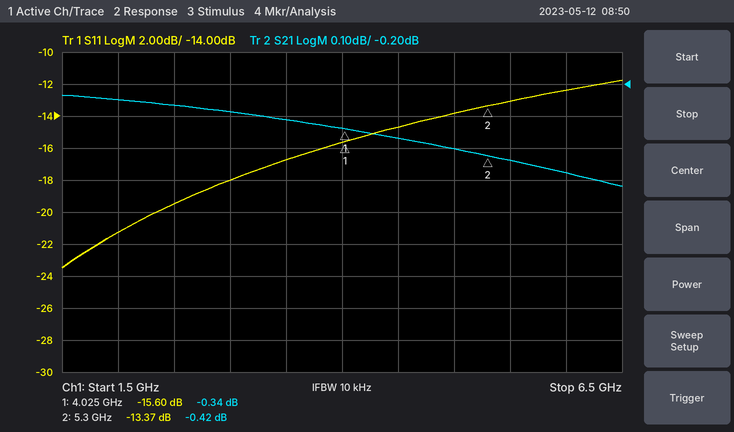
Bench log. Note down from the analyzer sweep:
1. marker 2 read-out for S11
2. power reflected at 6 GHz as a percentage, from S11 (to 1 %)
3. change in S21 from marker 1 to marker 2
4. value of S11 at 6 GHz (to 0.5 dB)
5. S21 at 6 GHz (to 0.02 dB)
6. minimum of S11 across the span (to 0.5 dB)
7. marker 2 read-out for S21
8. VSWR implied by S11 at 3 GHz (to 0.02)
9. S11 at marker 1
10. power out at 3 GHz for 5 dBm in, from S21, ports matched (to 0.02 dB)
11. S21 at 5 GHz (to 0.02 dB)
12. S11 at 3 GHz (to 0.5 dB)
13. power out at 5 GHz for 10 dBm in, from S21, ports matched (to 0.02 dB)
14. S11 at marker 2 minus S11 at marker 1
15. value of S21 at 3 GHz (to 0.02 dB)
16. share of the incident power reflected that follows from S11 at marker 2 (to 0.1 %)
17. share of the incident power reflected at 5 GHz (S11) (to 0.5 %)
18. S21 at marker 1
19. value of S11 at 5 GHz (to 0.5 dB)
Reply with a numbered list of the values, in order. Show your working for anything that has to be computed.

1. -13.37 dB
2. 10^(-12.5/10) ≈ 6 %
3. -0.42 − (-0.34) = -0.08 dB
4. -12.5 dB
5. -0.48 dB
6. -23.5 dB
7. -0.42 dB
8. |Γ| = 10^(-18/20) = 0.1259; VSWR = (1 + 0.1259)/(1 − 0.1259) ≈ 1.29, so 1.28 to the nearest 0.02
9. -15.60 dB
10. 5 dBm + (-0.28 dB) = 4.72 dBm
11. -0.40 dB
12. -18.0 dB
13. 10 dBm + (-0.40 dB) = 9.60 dBm
14. -13.37 − (-15.6) = 2.23 dB
15. -0.28 dB
16. 10^(-13.37/10) ≈ 4.6 %
17. 10^(-14/10) ≈ 4.0 %
18. -0.34 dB
19. -14.0 dB
